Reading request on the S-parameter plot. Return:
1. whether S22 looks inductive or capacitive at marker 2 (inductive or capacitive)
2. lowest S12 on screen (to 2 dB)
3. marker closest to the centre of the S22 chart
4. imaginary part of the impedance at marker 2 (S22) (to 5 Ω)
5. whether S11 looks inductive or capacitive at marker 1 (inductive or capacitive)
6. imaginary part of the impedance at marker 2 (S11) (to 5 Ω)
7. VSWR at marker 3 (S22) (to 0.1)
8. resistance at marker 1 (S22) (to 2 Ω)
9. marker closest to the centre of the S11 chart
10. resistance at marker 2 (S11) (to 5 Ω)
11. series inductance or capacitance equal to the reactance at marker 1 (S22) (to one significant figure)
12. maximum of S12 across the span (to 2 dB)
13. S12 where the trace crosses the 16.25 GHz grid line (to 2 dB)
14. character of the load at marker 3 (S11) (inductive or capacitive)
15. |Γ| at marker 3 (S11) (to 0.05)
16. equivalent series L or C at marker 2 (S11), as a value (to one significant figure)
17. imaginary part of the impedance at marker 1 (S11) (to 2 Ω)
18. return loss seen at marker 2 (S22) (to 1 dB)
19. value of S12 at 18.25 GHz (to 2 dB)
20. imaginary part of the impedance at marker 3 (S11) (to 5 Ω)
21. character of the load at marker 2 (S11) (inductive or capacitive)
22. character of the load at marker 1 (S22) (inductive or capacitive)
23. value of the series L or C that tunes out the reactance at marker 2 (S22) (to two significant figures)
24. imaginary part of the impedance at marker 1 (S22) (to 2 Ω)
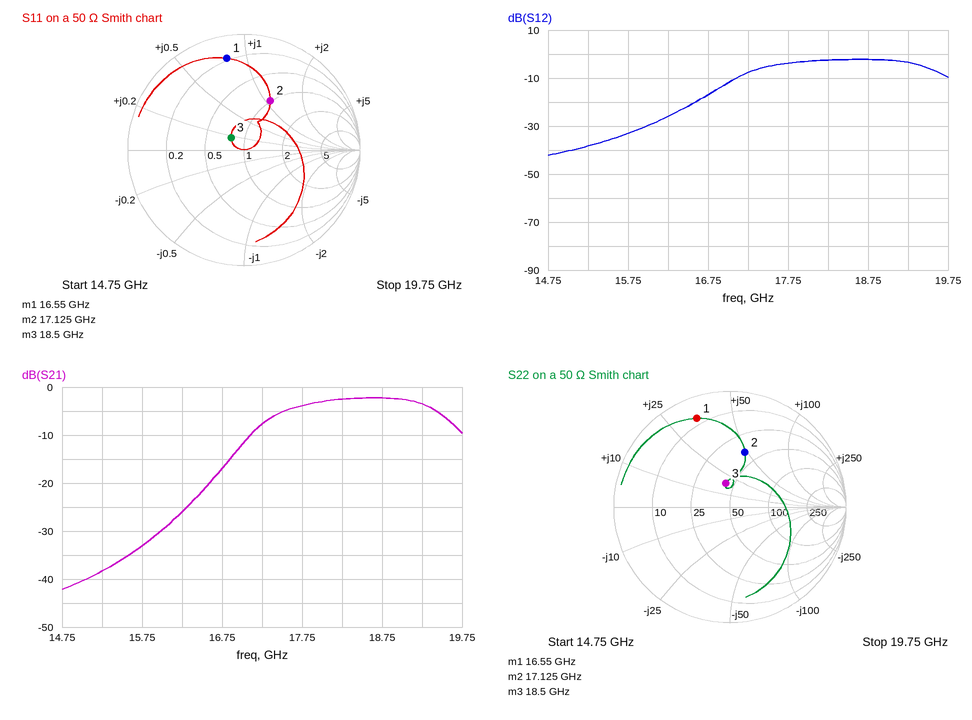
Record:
inductive
-42 dB
marker 3
+50 Ω
inductive
+55 Ω
1.5
8 Ω
marker 3
50 Ω
300 pH
-2 dB
-26 dB
inductive
0.15
500 pH
+40 Ω
6 dB
-2 dB
+10 Ω
inductive
inductive
190 fF
+34 Ω
